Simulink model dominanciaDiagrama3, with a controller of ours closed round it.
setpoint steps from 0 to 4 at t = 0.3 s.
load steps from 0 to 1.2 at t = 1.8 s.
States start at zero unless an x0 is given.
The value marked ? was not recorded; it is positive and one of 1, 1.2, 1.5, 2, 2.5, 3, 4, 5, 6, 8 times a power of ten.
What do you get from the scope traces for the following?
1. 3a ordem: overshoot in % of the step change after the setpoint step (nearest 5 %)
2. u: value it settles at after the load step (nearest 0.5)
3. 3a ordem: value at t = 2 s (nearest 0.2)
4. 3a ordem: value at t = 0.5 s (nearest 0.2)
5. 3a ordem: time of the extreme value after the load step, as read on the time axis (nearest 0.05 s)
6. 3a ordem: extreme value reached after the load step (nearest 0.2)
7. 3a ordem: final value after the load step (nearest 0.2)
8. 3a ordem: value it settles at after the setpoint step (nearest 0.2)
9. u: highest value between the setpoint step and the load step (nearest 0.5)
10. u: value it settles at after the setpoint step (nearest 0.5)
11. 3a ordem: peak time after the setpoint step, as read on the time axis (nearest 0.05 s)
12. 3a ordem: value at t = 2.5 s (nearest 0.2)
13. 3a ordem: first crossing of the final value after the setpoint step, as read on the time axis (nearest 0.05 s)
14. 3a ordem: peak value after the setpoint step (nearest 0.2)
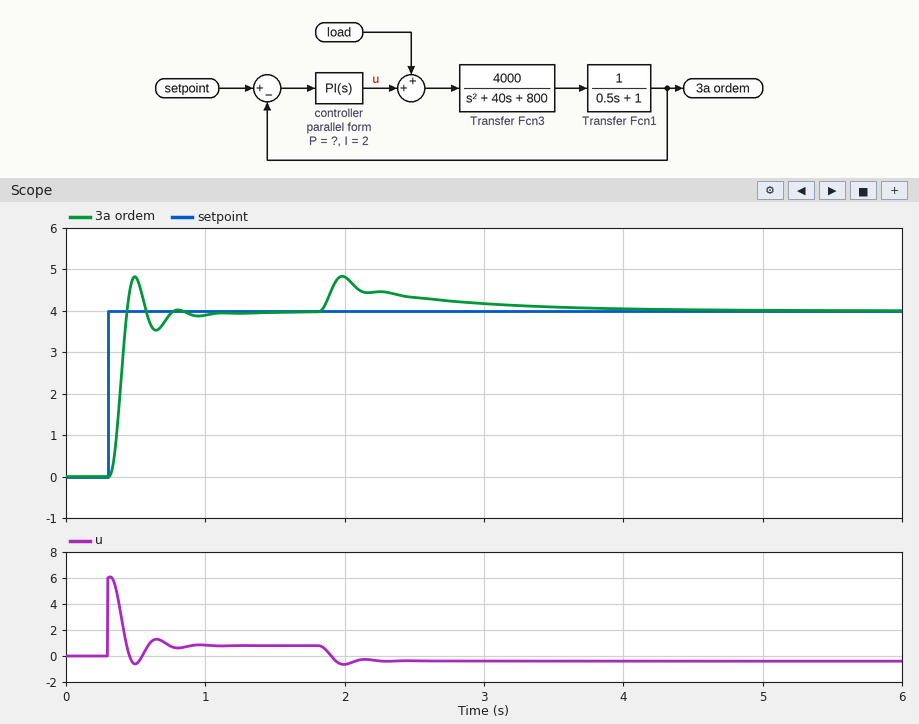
20 %
-0.5
4.8
4.8
2.00 s
4.8
4.0
4.0
6.0
1.0
0.50 s
4.4
0.45 s
4.8
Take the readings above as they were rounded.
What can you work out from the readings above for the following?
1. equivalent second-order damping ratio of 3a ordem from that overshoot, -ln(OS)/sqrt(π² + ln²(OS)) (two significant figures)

0.46
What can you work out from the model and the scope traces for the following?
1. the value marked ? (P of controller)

1.5
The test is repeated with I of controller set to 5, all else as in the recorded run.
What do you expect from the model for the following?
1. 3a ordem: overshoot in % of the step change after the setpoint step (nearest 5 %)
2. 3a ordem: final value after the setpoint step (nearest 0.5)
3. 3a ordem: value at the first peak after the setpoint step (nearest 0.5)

35 %
4.0
5.5
